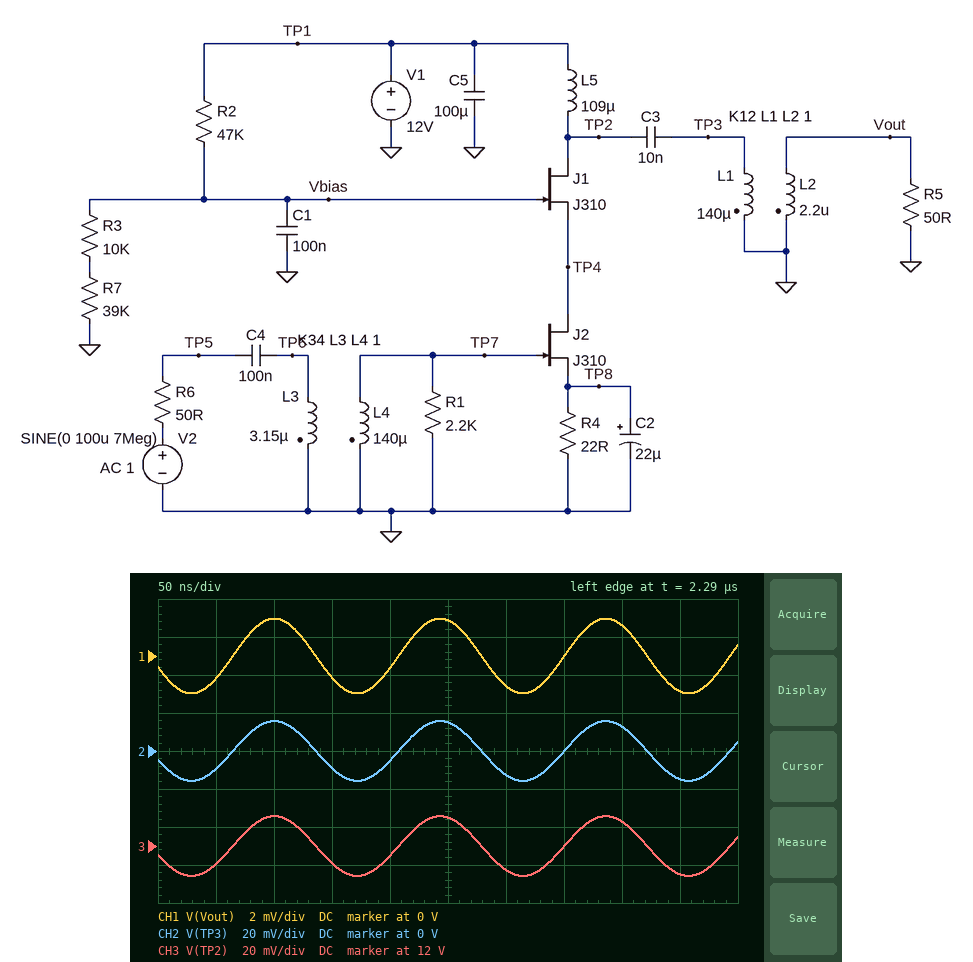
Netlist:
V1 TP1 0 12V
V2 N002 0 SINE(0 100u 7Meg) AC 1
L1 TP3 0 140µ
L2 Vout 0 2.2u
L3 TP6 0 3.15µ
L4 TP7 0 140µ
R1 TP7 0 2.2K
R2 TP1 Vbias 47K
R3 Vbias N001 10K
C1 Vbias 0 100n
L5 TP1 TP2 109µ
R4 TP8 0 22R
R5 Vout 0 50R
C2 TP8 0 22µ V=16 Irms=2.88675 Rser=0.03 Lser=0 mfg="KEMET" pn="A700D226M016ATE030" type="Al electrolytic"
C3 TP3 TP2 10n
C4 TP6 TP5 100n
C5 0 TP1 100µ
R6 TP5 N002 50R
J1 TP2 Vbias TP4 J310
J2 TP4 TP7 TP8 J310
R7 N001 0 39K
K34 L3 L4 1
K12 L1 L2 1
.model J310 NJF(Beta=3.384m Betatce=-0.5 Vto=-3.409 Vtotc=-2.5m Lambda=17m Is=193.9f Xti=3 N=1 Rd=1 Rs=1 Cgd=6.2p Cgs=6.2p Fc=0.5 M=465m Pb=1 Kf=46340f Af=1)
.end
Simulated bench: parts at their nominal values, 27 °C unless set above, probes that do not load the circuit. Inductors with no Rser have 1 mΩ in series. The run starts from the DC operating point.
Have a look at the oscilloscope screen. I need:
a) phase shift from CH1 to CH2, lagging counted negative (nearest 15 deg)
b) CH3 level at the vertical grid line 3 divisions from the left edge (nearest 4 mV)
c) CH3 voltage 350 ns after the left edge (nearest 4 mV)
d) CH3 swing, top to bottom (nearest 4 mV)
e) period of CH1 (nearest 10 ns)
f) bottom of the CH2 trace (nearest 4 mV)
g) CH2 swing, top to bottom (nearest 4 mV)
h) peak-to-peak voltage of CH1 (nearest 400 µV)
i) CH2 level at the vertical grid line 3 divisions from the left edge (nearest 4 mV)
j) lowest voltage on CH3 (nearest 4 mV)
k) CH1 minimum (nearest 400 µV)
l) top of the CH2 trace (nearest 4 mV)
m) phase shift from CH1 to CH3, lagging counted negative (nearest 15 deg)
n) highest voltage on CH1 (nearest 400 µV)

0 deg
11.992 V
12.000 V
32 mV
140 ns
-16 mV
32 mV
4.0 mV
-8 mV
11.984 V
-2.0 mV
16 mV
0 deg
2.0 mV
